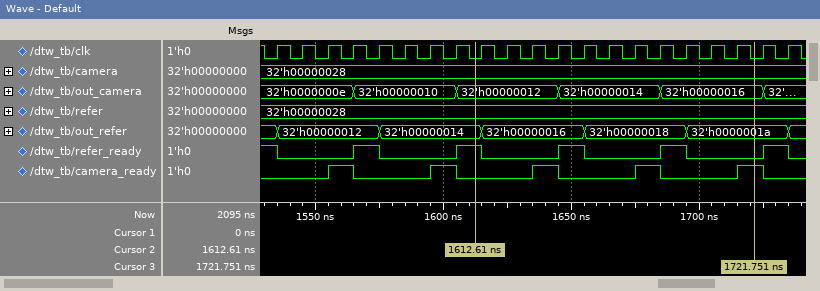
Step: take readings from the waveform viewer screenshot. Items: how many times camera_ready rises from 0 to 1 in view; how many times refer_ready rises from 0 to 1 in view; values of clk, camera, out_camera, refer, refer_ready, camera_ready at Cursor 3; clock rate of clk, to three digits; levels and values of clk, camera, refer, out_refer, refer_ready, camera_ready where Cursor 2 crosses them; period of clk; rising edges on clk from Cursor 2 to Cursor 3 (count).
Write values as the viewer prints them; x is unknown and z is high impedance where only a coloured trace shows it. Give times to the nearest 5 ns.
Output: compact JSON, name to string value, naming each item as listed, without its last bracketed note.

{"how many times camera_ready rises from 0 to 1 in view": "5", "how many times refer_ready rises from 0 to 1 in view": "5", "values of clk, camera, out_camera, refer, refer_ready, camera_ready at Cursor 3": "clk=0, camera=32'h00000028, out_camera=32'h00000016, refer=32'h00000028, refer_ready=0, camera_ready=1", "clock rate of clk, to three digits": "100 MHz", "levels and values of clk, camera, refer, out_refer, refer_ready, camera_ready where Cursor 2 crosses them": "clk=0, camera=32'h00000028, refer=32'h00000028, out_refer=32'h00000014, refer_ready=1, camera_ready=0", "period of clk": "10 ns", "rising edges on clk from Cursor 2 to Cursor 3": "11"}
